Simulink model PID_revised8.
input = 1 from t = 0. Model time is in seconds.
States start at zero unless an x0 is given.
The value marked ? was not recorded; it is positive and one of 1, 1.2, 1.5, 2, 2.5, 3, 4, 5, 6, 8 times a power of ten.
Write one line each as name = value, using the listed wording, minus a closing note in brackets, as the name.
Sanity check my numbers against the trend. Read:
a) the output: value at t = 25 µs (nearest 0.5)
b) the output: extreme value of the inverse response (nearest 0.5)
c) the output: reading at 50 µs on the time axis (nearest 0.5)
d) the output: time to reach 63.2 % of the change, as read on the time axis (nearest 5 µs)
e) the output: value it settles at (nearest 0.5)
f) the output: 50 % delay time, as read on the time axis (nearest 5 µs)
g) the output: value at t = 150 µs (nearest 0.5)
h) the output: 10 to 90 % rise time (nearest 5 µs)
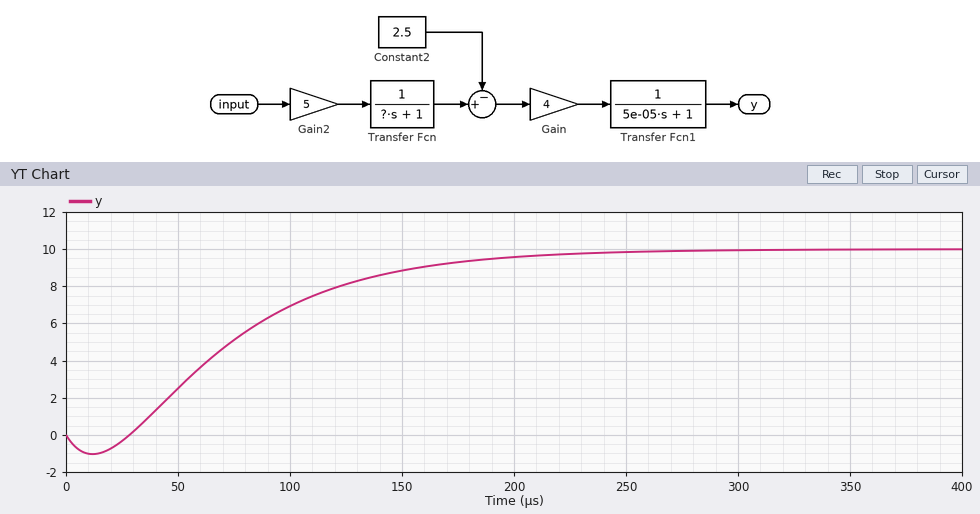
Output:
the output: value at t = 25 µs = -0.5
the output: extreme value of the inverse response = -1.0
the output: reading at 50 µs on the time axis = 2.5
the output: time to reach 63.2 % of the change, as read on the time axis = 90 µs
the output: value it settles at = 10.0
the output: 50 % delay time, as read on the time axis = 75 µs
the output: value at t = 150 µs = 9.0
the output: 10 to 90 % rise time = 120 µs
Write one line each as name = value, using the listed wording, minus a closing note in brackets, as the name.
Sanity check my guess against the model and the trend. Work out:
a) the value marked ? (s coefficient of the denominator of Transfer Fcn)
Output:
the value marked ? = 2e-05
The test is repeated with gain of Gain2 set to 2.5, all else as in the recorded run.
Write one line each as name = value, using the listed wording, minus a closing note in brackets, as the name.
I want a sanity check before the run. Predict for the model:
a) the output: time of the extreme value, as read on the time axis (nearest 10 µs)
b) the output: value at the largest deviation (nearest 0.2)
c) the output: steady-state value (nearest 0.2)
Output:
the output: time of the extreme value, as read on the time axis = 30 µs
the output: value at the largest deviation = -2.2
the output: steady-state value = 0.0
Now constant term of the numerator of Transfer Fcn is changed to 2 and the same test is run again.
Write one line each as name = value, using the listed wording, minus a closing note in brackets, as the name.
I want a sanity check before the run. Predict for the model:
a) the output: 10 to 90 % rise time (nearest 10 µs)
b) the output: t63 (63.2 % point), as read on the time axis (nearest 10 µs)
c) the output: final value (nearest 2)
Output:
the output: 10 to 90 % rise time = 120 µs
the output: t63 (63.2 % point), as read on the time axis = 80 µs
the output: final value = 30
